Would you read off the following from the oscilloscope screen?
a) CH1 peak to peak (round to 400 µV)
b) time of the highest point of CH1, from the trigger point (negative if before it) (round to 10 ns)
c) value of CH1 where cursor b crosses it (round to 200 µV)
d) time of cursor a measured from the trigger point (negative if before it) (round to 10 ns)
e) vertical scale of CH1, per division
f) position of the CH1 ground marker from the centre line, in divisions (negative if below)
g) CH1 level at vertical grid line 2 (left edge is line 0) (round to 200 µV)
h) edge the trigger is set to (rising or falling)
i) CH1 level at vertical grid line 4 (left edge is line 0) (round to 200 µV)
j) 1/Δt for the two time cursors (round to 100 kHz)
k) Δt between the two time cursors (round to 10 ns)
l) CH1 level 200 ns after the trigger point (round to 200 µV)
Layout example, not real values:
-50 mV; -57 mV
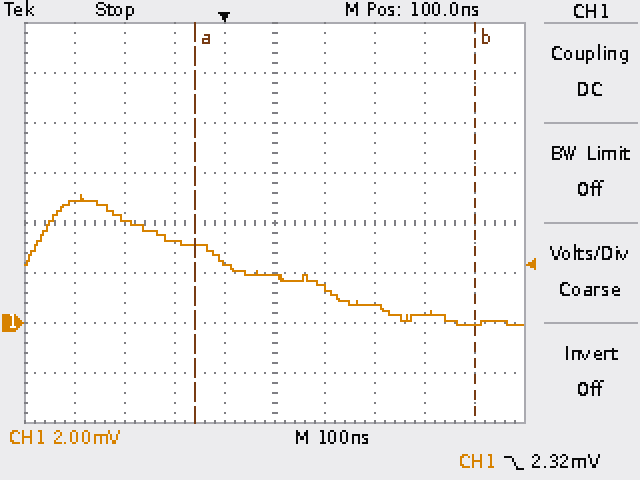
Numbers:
5.2 mV; -280 ns; 0.0 mV; -60 ns; 2 mV; -2.0 div; 4.2 mV; falling; 2.4 mV; 1.8 MHz; 560 ns; 1.4 mV
